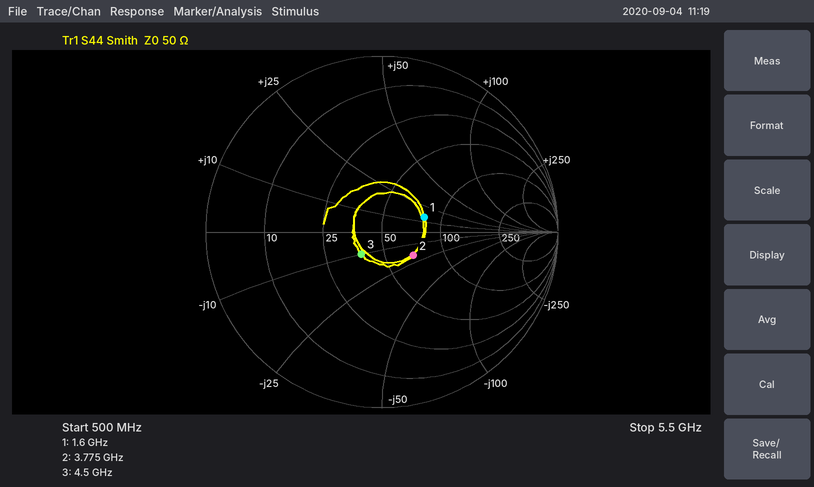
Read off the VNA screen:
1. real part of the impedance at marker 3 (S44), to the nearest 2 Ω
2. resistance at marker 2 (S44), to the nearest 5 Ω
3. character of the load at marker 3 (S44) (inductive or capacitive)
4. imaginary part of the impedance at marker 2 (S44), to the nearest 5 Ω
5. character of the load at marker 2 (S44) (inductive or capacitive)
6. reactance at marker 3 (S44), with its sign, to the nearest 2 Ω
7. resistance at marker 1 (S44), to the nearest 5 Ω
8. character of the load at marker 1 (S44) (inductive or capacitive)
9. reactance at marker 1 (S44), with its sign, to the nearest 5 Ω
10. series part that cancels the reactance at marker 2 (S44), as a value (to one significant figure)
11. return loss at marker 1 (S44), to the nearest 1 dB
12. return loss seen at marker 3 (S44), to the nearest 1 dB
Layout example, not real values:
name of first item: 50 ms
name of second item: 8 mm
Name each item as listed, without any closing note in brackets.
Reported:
real part of the impedance at marker 3 (S44), to the nearest 2 Ω: 38 Ω
resistance at marker 2 (S44), to the nearest 5 Ω: 70 Ω
character of the load at marker 3 (S44): capacitive
imaginary part of the impedance at marker 2 (S44), to the nearest 5 Ω: -20 Ω
character of the load at marker 2 (S44): capacitive
reactance at marker 3 (S44), with its sign, to the nearest 2 Ω: -10 Ω
resistance at marker 1 (S44), to the nearest 5 Ω: 80 Ω
character of the load at marker 1 (S44): inductive
reactance at marker 1 (S44), with its sign, to the nearest 5 Ω: +15 Ω
series part that cancels the reactance at marker 2 (S44), as a value: 800 pH
return loss at marker 1 (S44), to the nearest 1 dB: 12 dB
return loss seen at marker 3 (S44), to the nearest 1 dB: 15 dB
